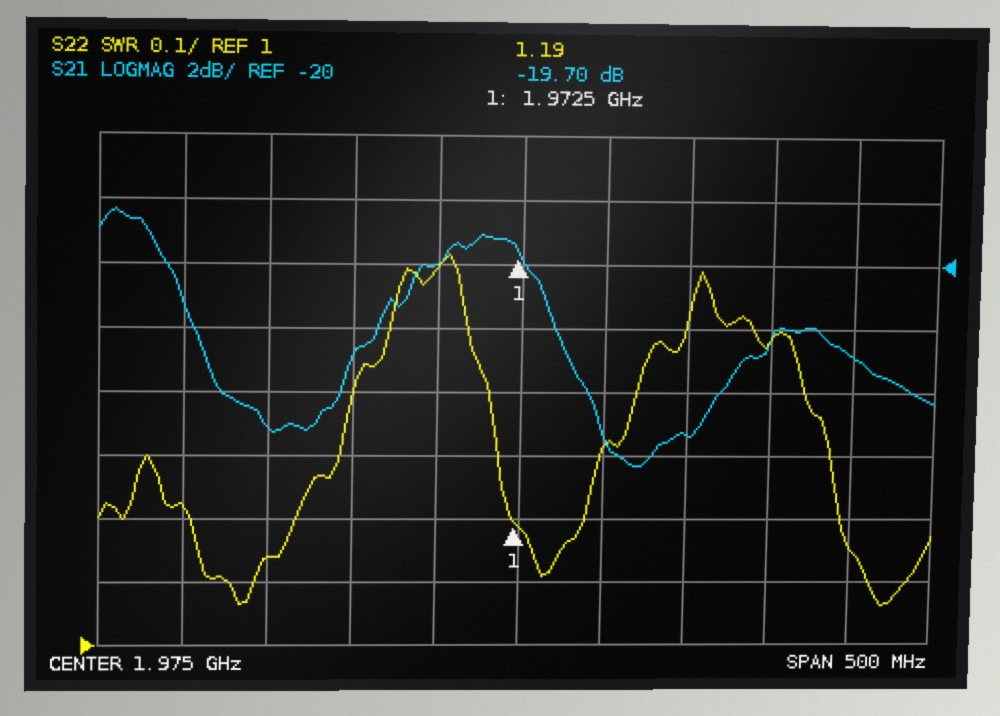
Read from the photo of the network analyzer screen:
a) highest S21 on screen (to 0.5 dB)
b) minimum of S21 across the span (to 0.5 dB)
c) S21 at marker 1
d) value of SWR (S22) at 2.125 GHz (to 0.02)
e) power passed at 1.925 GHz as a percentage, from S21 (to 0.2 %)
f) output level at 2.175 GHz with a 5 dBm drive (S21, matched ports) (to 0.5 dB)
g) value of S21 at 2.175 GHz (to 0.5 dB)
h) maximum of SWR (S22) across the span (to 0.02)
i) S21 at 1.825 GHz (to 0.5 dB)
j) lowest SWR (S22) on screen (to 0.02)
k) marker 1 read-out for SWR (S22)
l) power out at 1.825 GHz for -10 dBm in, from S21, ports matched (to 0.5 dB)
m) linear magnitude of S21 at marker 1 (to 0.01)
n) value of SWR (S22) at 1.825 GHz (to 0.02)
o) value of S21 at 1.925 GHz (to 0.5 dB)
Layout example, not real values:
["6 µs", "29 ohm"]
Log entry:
["-18.5 dB", "-26.5 dB", "-19.70 dB", "1.48", "1.0 %", "-18.0 dBm", "-23.0 dB", "1.62", "-25.0 dB", "1.06", "1.19", "-35.0 dBm", "0.10", "1.14", "-20.0 dB"]
